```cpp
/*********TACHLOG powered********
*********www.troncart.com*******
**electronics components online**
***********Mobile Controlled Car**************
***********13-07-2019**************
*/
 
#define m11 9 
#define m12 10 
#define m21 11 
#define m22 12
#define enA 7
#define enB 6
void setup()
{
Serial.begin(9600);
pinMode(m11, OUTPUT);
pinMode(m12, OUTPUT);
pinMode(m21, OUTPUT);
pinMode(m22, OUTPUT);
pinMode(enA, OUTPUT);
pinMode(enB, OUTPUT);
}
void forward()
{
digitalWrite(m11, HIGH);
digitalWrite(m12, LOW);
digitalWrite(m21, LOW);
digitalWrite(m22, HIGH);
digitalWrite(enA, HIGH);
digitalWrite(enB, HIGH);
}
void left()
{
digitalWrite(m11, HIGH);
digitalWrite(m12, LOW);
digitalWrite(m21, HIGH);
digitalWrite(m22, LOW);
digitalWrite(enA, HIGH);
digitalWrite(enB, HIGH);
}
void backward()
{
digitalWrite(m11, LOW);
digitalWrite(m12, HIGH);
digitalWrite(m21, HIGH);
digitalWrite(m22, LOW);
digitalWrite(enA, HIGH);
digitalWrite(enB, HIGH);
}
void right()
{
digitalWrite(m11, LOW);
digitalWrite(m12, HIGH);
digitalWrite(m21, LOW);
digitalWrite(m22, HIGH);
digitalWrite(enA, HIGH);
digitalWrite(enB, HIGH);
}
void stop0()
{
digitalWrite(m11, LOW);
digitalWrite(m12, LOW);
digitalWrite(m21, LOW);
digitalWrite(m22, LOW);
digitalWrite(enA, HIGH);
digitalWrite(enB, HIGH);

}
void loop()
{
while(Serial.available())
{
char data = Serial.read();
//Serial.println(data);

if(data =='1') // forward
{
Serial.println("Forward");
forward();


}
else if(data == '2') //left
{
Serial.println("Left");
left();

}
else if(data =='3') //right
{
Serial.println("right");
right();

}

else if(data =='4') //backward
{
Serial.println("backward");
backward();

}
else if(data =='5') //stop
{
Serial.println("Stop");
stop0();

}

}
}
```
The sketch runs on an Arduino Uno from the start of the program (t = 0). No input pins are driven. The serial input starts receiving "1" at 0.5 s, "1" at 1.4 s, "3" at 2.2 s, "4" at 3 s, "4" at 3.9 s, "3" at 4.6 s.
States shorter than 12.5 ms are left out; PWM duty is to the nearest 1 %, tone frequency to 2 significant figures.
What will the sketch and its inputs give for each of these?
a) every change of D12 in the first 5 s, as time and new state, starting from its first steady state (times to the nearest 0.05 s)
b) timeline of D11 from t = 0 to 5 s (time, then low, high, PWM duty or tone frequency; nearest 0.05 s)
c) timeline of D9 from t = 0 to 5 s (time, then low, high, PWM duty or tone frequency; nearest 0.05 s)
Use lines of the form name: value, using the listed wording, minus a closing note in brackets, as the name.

every change of D12 in the first 5 s, as time and new state, starting from its first steady state: 0 s low; 0.5 s high; 3 s low; 4.6 s high
timeline of D11 from t = 0 to 5 s: 0 s low; 3 s high; 4.6 s low
timeline of D9 from t = 0 to 5 s: 0 s low; 0.5 s high; 2.2 s low
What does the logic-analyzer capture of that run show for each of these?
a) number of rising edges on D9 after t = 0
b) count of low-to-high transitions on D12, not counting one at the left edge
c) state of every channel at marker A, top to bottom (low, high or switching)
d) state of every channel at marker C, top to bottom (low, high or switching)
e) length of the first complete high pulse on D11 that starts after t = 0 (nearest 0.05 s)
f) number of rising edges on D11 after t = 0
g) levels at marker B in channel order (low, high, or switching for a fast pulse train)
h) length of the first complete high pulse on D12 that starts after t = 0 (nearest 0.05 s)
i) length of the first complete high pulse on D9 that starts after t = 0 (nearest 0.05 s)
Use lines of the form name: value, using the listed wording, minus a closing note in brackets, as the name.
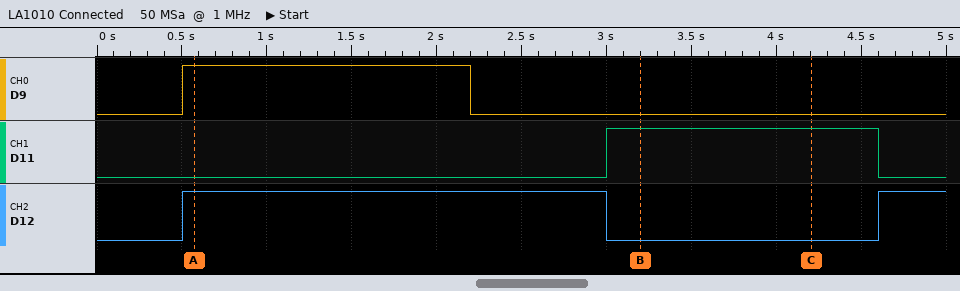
number of rising edges on D9 after t = 0: 1
count of low-to-high transitions on D12, not counting one at the left edge: 2
state of every channel at marker A, top to bottom: D9 high, D11 low, D12 high
state of every channel at marker C, top to bottom: D9 low, D11 high, D12 low
length of the first complete high pulse on D11 that starts after t = 0: 1.60 s
number of rising edges on D11 after t = 0: 1
levels at marker B in channel order: D9 low, D11 high, D12 low
length of the first complete high pulse on D12 that starts after t = 0: 2.50 s
length of the first complete high pulse on D9 that starts after t = 0: 1.70 s
